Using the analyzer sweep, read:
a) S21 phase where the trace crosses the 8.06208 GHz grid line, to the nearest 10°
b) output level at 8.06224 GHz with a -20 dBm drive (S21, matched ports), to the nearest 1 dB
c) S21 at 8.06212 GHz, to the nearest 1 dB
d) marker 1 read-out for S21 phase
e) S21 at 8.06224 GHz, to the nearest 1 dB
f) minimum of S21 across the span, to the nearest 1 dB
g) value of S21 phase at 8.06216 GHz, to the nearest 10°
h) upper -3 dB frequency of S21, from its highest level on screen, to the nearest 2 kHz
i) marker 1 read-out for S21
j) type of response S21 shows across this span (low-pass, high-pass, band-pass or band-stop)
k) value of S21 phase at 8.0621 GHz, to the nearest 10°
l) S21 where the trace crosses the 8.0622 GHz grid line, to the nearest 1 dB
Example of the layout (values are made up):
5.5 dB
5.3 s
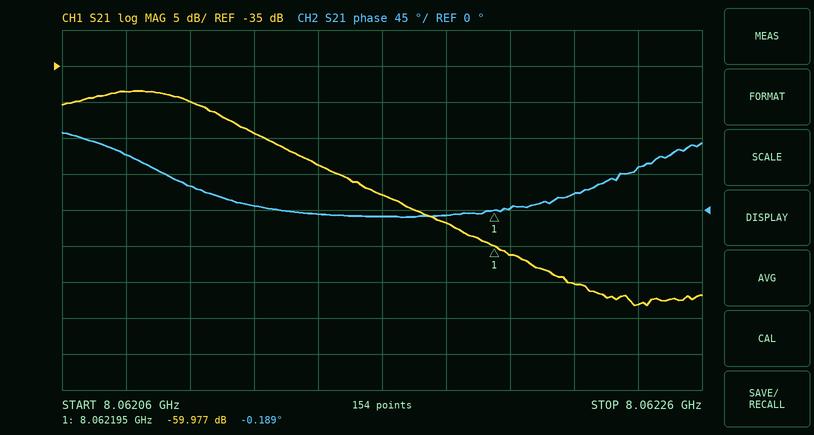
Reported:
70°
-88 dBm
-44 dB
-0.189°
-68 dB
-68 dB
-10°
8.062108 GHz
-59.977 dB
low-pass
30°
-61 dB
